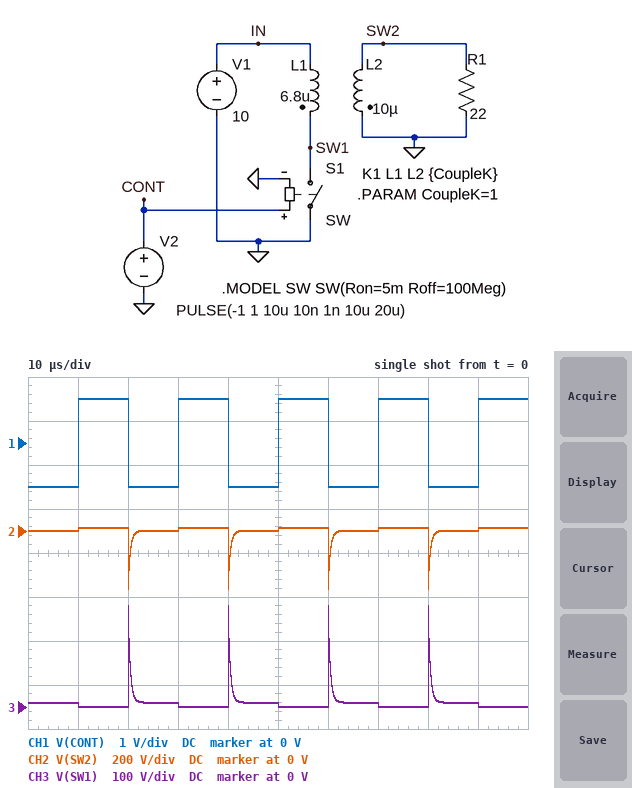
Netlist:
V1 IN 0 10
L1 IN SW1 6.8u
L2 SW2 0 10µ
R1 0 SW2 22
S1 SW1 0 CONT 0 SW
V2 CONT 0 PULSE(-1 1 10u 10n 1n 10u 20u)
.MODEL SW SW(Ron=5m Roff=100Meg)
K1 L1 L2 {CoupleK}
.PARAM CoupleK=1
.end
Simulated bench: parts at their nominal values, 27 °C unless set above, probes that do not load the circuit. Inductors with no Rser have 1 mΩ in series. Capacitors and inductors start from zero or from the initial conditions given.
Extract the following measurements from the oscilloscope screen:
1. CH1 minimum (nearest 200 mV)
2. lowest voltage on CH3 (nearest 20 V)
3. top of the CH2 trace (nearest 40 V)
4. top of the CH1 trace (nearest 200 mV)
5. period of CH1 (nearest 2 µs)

-1.0 V
0 V
0 V
1.0 V
20 µs
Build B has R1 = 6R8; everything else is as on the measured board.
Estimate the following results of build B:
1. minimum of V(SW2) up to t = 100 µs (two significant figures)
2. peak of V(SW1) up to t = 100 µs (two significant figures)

-82 V
78 V
